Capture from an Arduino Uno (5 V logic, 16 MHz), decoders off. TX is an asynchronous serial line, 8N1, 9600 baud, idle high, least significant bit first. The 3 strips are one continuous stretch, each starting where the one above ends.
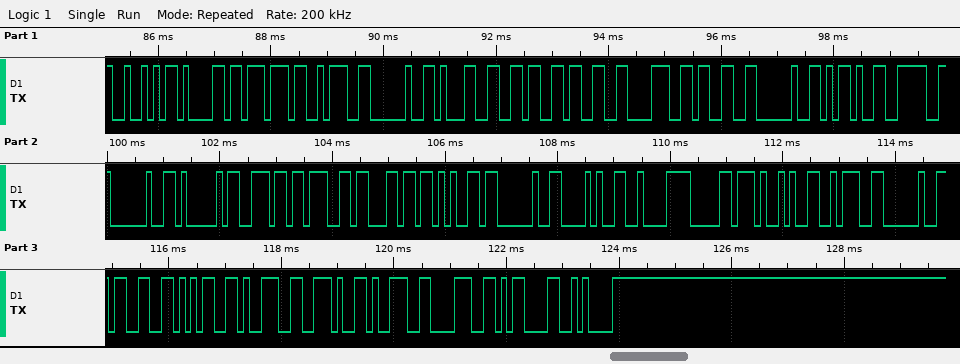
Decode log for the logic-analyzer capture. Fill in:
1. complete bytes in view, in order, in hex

52 61 77 3A 20 31 36 33 38 33 20 2D 3E 20 41 6E 67 6C 65 20 28 C2 B0 29 3A 20 33 35 39 2E 39 38 0D 0A
